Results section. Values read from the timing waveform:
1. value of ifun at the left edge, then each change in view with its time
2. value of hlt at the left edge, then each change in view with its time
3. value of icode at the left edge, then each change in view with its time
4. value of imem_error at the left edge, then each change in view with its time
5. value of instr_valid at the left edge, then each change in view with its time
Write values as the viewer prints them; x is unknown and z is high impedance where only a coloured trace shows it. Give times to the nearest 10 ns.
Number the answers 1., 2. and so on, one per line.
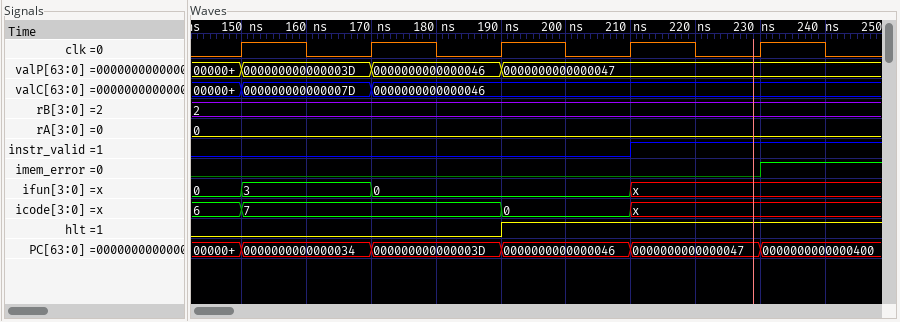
1. 0, 3 at 150 ns, 0 at 170 ns, x at 210 ns
2. 0, 1 at 190 ns
3. 6, 7 at 150 ns, 0 at 190 ns, x at 210 ns
4. 0, 1 at 230 ns
5. 0, 1 at 210 ns
